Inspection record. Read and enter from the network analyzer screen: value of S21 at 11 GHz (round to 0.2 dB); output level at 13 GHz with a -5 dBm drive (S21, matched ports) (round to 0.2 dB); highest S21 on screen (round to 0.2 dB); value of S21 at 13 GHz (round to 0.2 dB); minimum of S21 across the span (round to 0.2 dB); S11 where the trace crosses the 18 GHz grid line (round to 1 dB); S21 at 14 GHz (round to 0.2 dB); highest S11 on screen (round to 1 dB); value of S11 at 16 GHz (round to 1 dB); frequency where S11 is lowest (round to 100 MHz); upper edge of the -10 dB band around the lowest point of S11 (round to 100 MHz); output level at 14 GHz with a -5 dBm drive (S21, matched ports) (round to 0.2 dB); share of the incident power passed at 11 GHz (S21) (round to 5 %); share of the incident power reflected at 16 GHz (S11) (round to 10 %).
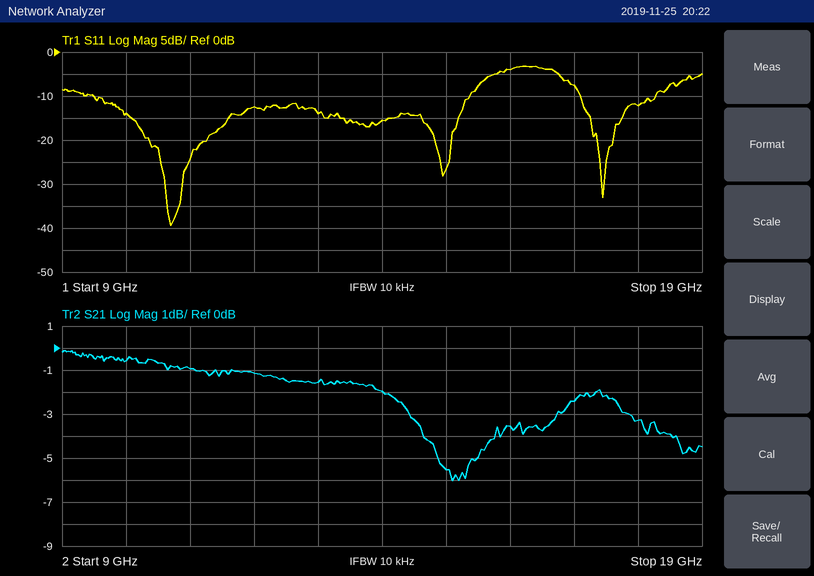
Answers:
-1.0 dB
-6.6 dBm
-0.2 dB
-1.6 dB
-6.0 dB
-12 dB
-2.0 dB
-3 dB
-4 dB
10.7 GHz
15.4 GHz
-7.0 dBm
80 %
40 %
